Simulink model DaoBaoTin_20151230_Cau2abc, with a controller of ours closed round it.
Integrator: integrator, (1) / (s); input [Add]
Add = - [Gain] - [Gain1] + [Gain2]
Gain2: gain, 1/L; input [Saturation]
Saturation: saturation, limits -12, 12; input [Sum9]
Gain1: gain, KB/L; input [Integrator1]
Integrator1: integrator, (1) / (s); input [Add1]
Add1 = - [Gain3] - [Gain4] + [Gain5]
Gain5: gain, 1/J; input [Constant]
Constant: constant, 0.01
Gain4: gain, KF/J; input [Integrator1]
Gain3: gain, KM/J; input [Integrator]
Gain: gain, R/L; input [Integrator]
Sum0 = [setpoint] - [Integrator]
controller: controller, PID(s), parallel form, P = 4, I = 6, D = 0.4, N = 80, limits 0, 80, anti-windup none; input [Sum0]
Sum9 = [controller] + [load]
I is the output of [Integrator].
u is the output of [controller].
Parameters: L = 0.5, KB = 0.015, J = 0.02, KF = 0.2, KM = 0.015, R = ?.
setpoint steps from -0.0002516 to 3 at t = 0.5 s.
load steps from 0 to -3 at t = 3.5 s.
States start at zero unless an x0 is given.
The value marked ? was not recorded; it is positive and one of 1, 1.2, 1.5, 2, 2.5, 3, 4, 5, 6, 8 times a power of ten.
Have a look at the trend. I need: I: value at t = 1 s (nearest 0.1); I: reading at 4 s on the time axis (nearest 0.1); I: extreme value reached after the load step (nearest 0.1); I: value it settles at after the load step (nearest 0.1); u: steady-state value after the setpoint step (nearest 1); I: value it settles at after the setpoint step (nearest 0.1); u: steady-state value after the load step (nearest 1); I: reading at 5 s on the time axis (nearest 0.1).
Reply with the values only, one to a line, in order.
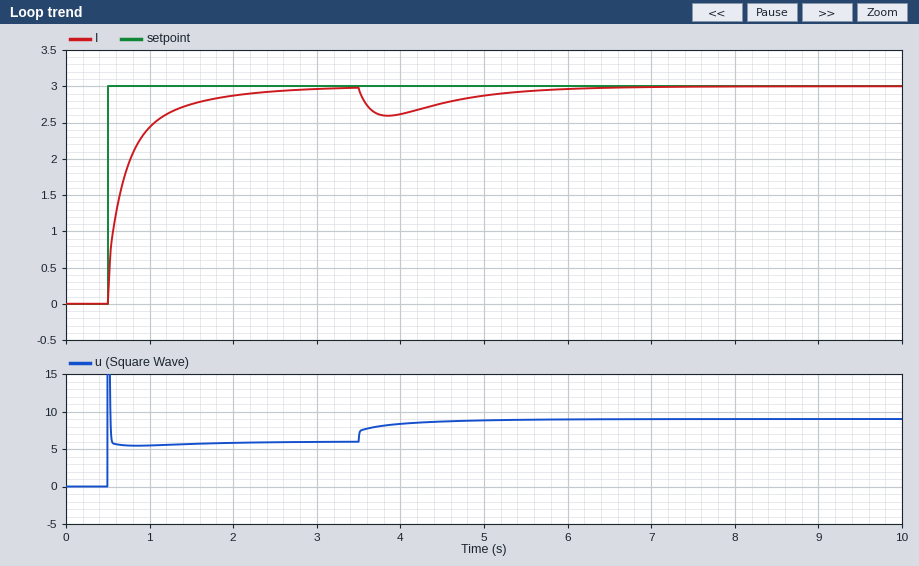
2.4
2.6
2.6
3.0
6
3.0
9
2.9
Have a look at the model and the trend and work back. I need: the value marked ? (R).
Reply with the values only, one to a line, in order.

2
